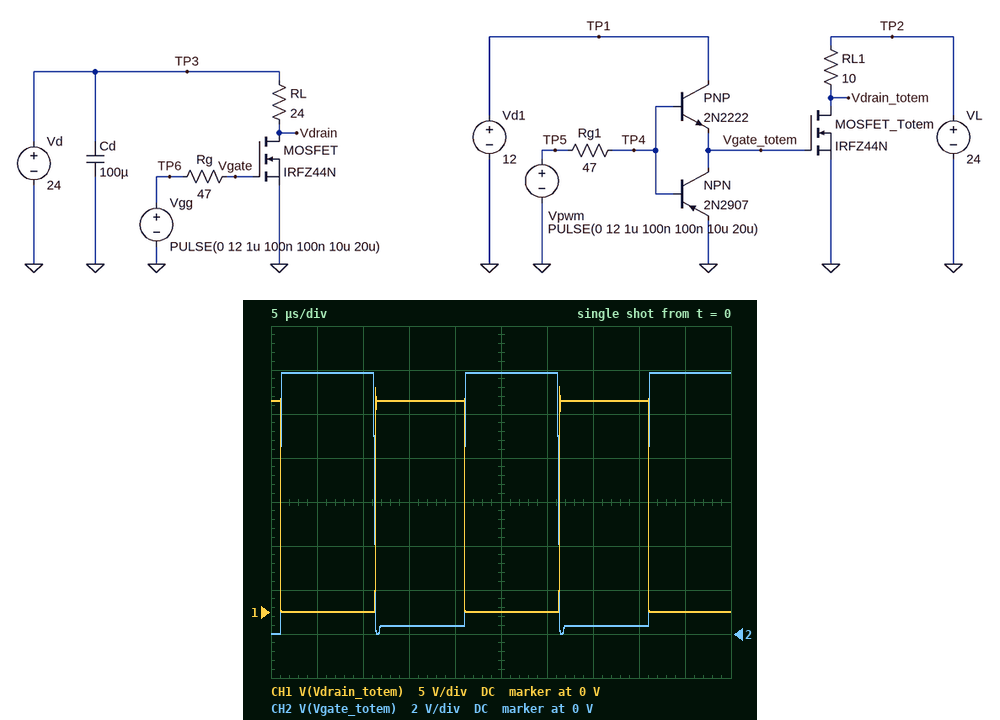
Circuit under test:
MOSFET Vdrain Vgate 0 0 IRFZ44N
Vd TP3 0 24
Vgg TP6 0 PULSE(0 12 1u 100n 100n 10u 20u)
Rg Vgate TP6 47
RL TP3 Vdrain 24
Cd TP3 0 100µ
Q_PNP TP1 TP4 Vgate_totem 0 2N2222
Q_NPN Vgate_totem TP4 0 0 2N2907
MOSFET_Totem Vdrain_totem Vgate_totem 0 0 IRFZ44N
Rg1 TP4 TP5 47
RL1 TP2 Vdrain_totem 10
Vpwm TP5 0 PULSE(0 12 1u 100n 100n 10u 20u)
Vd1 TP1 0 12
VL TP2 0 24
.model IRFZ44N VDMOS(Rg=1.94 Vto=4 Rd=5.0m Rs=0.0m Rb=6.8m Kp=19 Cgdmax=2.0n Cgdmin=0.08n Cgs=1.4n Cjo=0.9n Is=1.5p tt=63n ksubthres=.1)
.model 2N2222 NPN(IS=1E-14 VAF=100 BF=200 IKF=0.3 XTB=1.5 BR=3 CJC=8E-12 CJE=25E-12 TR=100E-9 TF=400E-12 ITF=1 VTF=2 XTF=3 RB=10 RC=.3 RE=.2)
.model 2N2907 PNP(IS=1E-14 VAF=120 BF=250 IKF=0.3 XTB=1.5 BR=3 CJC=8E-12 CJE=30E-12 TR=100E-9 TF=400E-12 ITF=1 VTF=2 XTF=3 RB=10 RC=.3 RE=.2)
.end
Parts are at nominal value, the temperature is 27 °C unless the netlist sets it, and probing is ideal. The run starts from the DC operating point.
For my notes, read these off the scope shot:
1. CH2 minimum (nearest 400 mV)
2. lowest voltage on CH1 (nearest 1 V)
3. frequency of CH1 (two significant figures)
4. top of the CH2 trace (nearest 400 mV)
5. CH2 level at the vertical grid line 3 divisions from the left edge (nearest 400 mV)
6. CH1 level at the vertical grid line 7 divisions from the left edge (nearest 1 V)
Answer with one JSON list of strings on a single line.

["0 V", "0 V", "50 kHz", "12.0 V", "400 mV", "24 V"]
